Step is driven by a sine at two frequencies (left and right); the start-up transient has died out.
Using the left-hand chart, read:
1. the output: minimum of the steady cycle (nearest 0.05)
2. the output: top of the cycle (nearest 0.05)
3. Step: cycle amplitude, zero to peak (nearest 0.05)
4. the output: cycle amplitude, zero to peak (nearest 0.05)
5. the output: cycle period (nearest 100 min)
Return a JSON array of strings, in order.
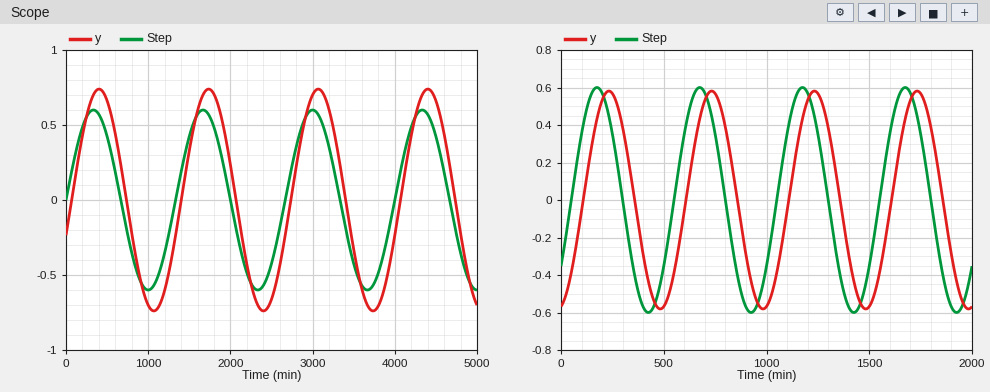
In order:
["-0.75", "0.75", "0.60", "0.75", "1300 min"]
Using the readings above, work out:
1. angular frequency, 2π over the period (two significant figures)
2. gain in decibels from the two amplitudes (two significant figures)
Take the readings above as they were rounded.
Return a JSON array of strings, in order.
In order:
["0.0048 rad/min", "1.9 dB"]
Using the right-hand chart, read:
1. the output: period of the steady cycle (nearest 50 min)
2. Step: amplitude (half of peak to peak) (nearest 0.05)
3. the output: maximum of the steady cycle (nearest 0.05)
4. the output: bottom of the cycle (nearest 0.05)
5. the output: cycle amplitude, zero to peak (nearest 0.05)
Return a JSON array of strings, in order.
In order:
["500 min", "0.60", "0.60", "-0.60", "0.60"]
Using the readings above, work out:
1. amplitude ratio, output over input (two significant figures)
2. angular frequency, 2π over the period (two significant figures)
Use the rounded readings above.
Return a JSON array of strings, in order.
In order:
["1.0", "0.013 rad/min"]
